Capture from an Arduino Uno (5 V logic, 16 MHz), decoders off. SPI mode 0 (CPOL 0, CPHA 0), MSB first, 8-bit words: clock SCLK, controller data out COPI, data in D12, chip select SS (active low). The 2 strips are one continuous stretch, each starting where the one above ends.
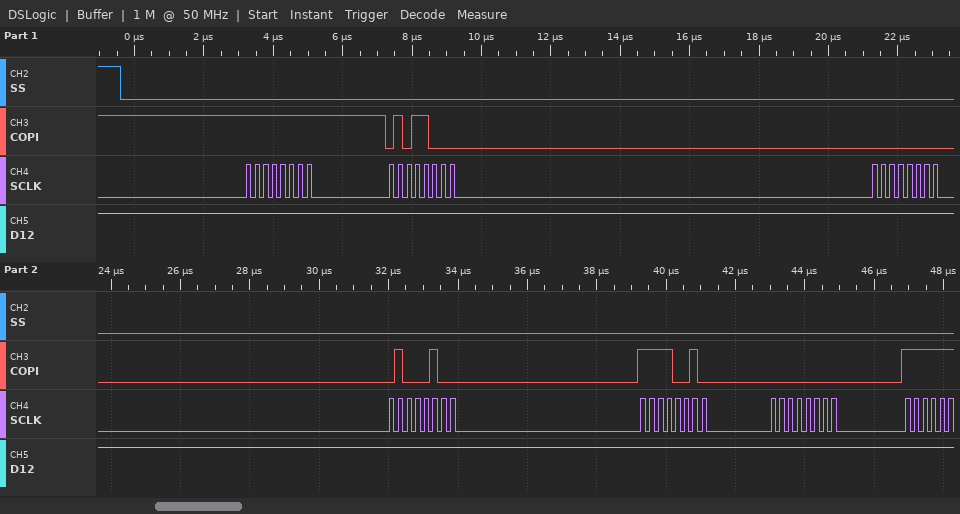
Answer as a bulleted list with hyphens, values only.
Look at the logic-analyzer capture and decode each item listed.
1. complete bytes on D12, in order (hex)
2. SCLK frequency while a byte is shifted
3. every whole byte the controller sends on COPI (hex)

- FF FF FF FF FF FF
- 4 MHz
- FF 58 00 44 F2 00
